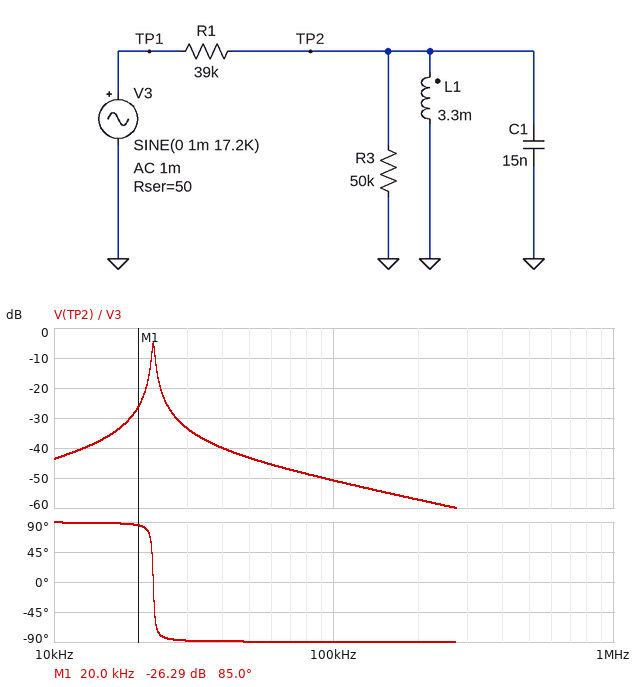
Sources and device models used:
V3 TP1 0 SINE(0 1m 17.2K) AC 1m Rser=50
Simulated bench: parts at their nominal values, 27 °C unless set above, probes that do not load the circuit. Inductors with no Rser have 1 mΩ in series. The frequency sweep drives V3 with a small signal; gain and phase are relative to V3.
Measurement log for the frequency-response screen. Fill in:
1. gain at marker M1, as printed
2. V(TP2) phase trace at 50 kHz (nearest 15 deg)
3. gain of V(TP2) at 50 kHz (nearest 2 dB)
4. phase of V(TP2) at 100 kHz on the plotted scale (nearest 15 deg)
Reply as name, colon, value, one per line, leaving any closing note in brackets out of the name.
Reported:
gain at marker M1, as printed: -26.29 dB
V(TP2) phase trace at 50 kHz: -90 deg
gain of V(TP2) at 50 kHz: -44 dB
phase of V(TP2) at 100 kHz on the plotted scale: -90 deg
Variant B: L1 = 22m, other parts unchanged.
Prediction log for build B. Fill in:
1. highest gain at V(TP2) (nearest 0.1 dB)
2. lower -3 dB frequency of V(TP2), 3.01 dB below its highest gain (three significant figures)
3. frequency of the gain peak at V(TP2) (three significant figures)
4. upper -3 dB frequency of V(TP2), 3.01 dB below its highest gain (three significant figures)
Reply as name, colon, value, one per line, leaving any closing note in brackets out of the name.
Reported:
highest gain at V(TP2): -5.0 dB
lower -3 dB frequency of V(TP2), 3.01 dB below its highest gain: 8.52 kHz
frequency of the gain peak at V(TP2): 8.76 kHz
upper -3 dB frequency of V(TP2), 3.01 dB below its highest gain: 9.01 kHz
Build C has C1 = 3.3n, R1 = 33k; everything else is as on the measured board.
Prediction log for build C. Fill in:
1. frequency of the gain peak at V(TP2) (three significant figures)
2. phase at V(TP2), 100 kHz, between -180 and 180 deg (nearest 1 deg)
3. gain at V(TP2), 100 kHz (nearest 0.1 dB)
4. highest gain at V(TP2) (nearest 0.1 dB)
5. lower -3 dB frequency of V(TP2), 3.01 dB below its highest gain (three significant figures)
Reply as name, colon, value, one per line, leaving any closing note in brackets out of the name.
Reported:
frequency of the gain peak at V(TP2): 48.2 kHz
phase at V(TP2), 100 kHz, between -180 and 180 deg: -88 deg
gain at V(TP2), 100 kHz: -34.4 dB
highest gain at V(TP2): -4.4 dB
lower -3 dB frequency of V(TP2), 3.01 dB below its highest gain: 47.0 kHz
